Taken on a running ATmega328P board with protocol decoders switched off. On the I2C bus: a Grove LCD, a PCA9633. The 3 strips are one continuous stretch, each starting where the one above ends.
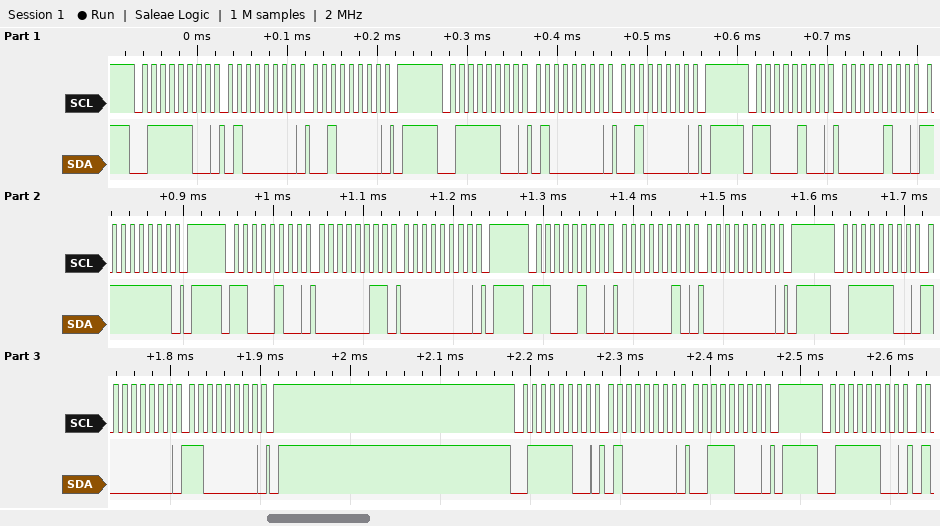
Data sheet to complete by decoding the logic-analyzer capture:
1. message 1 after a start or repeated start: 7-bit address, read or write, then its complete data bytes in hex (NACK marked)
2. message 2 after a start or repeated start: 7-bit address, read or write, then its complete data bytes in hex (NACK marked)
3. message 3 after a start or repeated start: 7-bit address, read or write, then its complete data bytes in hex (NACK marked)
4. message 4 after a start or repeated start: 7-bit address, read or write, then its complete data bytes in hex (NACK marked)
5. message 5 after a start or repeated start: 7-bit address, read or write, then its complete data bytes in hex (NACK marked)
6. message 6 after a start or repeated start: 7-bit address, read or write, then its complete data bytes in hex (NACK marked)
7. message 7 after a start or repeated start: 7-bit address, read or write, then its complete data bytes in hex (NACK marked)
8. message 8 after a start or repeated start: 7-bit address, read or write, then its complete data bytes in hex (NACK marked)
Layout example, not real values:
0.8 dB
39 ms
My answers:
0x3E write: 40 20
0x3E write: 40 20
0x62 write: 04 FF
0x62 write: 03 00
0x62 write: 02 00
0x3E write: 80 C0
0x3E write: 40 38
0x3E write
